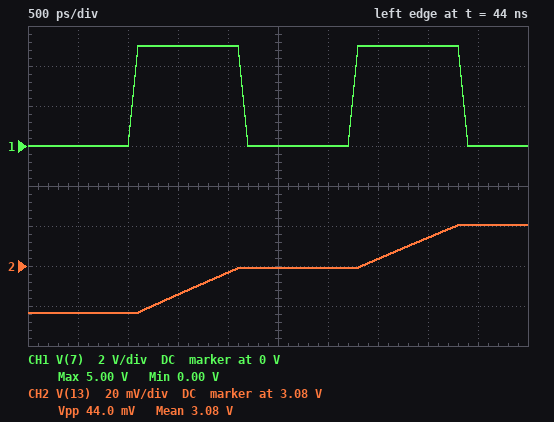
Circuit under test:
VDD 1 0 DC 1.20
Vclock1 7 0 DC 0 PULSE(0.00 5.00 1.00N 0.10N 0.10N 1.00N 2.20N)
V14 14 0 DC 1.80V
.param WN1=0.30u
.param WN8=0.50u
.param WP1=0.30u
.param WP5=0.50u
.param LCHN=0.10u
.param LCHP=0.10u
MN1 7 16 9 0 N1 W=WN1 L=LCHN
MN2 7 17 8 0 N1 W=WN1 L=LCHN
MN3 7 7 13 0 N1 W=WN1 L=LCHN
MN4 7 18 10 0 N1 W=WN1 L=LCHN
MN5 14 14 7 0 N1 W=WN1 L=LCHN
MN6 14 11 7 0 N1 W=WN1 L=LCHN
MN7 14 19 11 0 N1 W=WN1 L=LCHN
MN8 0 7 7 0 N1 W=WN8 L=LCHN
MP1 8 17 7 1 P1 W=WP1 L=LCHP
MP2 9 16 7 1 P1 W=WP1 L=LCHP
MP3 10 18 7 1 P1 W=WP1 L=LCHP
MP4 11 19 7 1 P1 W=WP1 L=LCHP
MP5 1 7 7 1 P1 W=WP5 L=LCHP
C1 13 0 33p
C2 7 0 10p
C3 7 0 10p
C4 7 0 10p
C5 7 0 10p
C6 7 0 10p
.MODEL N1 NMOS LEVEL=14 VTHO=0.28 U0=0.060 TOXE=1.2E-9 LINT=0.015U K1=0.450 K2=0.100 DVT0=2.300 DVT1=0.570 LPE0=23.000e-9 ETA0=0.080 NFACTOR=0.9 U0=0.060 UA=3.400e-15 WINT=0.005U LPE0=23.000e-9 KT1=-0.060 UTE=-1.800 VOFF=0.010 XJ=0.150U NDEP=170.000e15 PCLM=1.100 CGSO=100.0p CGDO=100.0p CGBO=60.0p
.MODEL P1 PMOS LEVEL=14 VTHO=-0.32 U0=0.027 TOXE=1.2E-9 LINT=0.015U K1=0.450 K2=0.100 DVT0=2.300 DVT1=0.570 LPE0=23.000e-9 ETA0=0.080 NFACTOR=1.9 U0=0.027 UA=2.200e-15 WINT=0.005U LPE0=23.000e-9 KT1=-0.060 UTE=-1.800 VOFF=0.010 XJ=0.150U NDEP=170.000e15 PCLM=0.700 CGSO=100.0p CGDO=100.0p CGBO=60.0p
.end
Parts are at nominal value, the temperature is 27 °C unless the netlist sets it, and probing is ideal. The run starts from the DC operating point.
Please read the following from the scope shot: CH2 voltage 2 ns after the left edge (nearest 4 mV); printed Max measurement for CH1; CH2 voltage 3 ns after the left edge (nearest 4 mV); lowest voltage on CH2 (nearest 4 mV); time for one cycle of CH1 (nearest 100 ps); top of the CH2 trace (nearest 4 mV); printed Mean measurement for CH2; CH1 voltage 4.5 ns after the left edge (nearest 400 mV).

3.076 V
5.00 V
3.080 V
3.056 V
2.2 ns
3.100 V
3.08 V
0 V
